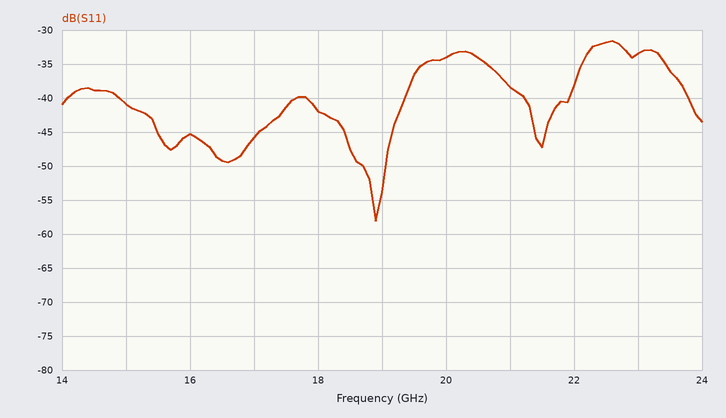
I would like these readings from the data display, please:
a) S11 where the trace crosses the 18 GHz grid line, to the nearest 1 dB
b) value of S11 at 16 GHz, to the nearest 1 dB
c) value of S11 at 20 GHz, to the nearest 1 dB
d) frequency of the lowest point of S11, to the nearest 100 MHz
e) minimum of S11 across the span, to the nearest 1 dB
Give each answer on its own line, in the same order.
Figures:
-42 dB
-45 dB
-34 dB
18.9 GHz
-58 dB
